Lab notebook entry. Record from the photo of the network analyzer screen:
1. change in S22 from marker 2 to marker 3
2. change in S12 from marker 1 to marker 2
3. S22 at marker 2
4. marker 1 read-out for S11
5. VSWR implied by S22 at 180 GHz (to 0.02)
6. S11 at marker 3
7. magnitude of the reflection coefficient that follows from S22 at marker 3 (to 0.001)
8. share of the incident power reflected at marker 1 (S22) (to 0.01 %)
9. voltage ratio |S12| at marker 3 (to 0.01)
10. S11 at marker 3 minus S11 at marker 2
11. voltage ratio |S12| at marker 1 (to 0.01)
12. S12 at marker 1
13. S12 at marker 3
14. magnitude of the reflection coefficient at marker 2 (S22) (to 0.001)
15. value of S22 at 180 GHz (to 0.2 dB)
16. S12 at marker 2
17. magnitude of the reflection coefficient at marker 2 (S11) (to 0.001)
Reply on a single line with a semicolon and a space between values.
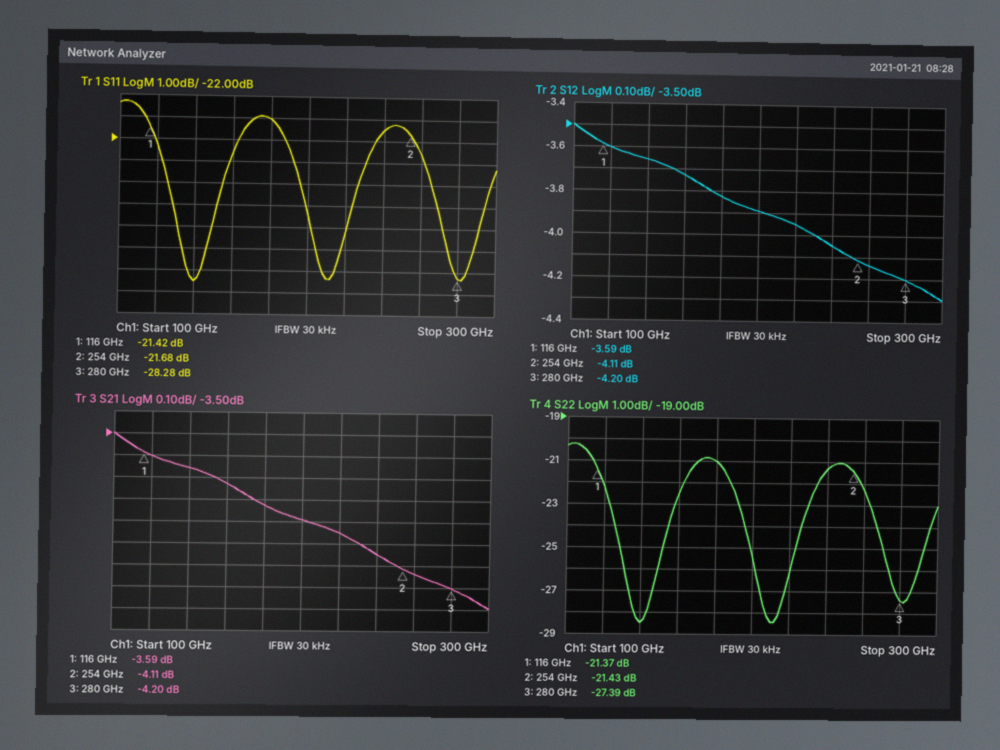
-5.96 dB; -0.52 dB; -21.43 dB; -21.42 dB; 1.20; -28.28 dB; 0.043; 0.73 %; 0.62; -6.60 dB; 0.66; -3.59 dB; -4.20 dB; 0.085; -21.0 dB; -4.11 dB; 0.082
